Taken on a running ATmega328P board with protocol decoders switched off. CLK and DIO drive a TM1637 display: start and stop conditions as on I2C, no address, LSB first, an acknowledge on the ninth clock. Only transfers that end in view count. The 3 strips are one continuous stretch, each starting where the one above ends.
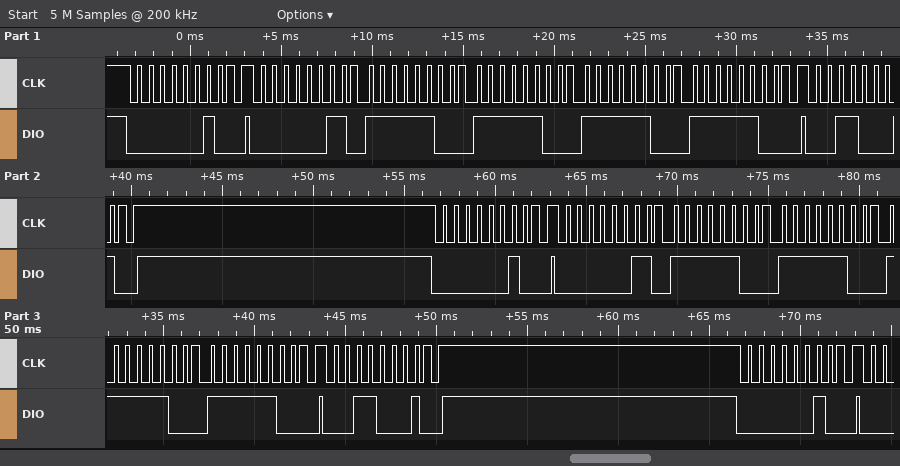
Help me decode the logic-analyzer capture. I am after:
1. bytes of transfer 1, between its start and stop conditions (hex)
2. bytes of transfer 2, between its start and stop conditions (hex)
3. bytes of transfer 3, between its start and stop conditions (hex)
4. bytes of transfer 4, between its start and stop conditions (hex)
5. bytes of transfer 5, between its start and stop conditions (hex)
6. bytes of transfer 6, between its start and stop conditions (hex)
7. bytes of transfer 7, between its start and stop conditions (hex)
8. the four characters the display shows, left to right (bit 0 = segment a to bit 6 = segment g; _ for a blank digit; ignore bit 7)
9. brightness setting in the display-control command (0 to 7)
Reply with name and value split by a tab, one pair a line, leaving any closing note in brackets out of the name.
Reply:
bytes of transfer 1, between its start and stop conditions	40
bytes of transfer 2, between its start and stop conditions	C0 3F 3F 3F 3F
bytes of transfer 3, between its start and stop conditions	8C
bytes of transfer 4, between its start and stop conditions	40
bytes of transfer 5, between its start and stop conditions	C0 3F 3F 3F 3F
bytes of transfer 6, between its start and stop conditions	8C
bytes of transfer 7, between its start and stop conditions	40
the four characters the display shows, left to right	0000
brightness setting in the display-control command	4
